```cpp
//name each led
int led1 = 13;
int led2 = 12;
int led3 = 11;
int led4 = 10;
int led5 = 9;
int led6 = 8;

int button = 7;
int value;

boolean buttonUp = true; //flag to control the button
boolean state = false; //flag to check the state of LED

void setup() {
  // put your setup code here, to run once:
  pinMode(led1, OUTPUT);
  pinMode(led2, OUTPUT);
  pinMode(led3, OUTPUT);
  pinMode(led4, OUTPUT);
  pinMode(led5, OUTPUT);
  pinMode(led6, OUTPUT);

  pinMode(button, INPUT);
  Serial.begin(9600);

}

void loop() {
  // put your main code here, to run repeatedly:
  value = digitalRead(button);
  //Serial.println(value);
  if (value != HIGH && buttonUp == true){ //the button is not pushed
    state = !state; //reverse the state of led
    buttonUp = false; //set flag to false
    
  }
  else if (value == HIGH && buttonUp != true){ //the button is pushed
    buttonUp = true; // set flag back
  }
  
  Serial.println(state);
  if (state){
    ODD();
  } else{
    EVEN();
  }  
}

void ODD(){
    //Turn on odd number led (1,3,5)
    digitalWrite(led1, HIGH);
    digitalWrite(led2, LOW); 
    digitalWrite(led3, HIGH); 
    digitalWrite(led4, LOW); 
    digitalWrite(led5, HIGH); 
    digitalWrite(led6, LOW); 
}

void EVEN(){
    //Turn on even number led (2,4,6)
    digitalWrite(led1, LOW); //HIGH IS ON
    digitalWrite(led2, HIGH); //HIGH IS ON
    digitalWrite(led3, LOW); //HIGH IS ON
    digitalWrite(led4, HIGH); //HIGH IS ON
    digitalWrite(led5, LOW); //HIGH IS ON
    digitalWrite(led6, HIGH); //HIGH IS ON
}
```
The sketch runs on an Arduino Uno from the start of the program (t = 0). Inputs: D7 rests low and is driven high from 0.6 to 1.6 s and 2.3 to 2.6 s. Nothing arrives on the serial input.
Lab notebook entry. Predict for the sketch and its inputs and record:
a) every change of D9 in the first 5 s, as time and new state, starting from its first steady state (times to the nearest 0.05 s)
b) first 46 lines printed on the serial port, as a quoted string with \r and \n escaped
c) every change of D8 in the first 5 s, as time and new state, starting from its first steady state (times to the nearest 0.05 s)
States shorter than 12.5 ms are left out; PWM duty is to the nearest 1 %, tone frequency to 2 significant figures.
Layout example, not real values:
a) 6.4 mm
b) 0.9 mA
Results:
a) 0 s high; 1.6 s low; 2.6 s high
b) "1\r\n1\r\n1\r\n1\r\n1\r\n1\r\n1\r\n1\r\n1\r\n1\r\n1\r\n1\r\n1\r\n1\r\n1\r\n1\r\n1\r\n1\r\n1\r\n1\r\n1\r\n1\r\n1\r\n1\r\n1\r\n1\r\n1\r\n1\r\n1\r\n1\r\n1\r\n1\r\n1\r\n1\r\n1\r\n1\r\n1\r\n1\r\n1\r\n1\r\n1\r\n1\r\n1\r\n1\r\n1\r\n1\r\n"
c) 0 s low; 1.6 s high; 2.6 s low
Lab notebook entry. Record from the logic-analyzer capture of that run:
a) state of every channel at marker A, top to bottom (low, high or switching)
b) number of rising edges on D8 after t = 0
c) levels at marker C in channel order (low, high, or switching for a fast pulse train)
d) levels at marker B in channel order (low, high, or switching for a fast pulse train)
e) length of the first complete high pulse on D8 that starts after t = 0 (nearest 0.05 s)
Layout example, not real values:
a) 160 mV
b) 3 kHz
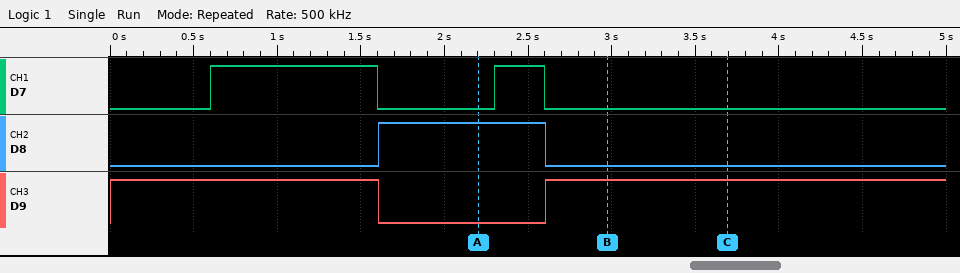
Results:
a) D7 low, D8 high, D9 low
b) 1
c) D7 low, D8 low, D9 high
d) D7 low, D8 low, D9 high
e) 1.00 s
